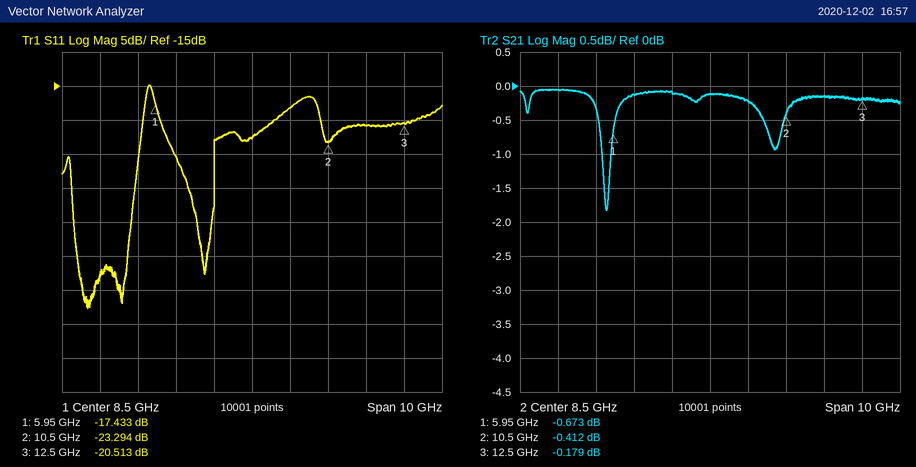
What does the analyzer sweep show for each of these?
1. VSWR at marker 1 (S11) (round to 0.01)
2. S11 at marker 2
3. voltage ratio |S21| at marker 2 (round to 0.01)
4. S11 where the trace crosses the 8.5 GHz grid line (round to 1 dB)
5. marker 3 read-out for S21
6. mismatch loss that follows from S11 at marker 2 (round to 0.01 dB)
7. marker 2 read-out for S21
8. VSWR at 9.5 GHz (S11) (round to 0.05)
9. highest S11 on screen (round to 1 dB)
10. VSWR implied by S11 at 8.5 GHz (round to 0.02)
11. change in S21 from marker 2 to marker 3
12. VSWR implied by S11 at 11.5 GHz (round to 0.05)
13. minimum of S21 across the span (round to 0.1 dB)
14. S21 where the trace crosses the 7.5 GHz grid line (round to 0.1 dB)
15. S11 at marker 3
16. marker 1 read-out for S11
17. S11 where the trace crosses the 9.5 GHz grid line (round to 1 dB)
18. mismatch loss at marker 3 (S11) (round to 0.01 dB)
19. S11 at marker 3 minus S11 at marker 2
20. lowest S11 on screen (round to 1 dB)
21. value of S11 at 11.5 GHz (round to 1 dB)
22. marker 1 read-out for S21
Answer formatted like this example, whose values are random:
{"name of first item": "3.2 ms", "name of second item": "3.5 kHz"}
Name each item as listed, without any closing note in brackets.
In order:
{"VSWR at marker 1 (S11)": "1.31", "S11 at marker 2": "-23.294 dB", "voltage ratio |S21| at marker 2": "0.95", "S11 where the trace crosses the 8.5 GHz grid line": "-23 dB", "marker 3 read-out for S21": "-0.179 dB", "mismatch loss that follows from S11 at marker 2": "0.02 dB", "marker 2 read-out for S21": "-0.412 dB", "VSWR at 9.5 GHz (S11)": "1.30", "highest S11 on screen": "-15 dB", "VSWR implied by S11 at 8.5 GHz": "1.16", "change in S21 from marker 2 to marker 3": "0.233 dB", "VSWR implied by S11 at 11.5 GHz": "1.20", "minimum of S21 across the span": "-1.8 dB", "S21 where the trace crosses the 7.5 GHz grid line": "-0.1 dB", "S11 at marker 3": "-20.513 dB", "marker 1 read-out for S11": "-17.433 dB", "S11 where the trace crosses the 9.5 GHz grid line": "-18 dB", "mismatch loss at marker 3 (S11)": "0.04 dB", "S11 at marker 3 minus S11 at marker 2": "2.781 dB", "lowest S11 on screen": "-48 dB", "value of S11 at 11.5 GHz": "-21 dB", "marker 1 read-out for S21": "-0.673 dB"}
